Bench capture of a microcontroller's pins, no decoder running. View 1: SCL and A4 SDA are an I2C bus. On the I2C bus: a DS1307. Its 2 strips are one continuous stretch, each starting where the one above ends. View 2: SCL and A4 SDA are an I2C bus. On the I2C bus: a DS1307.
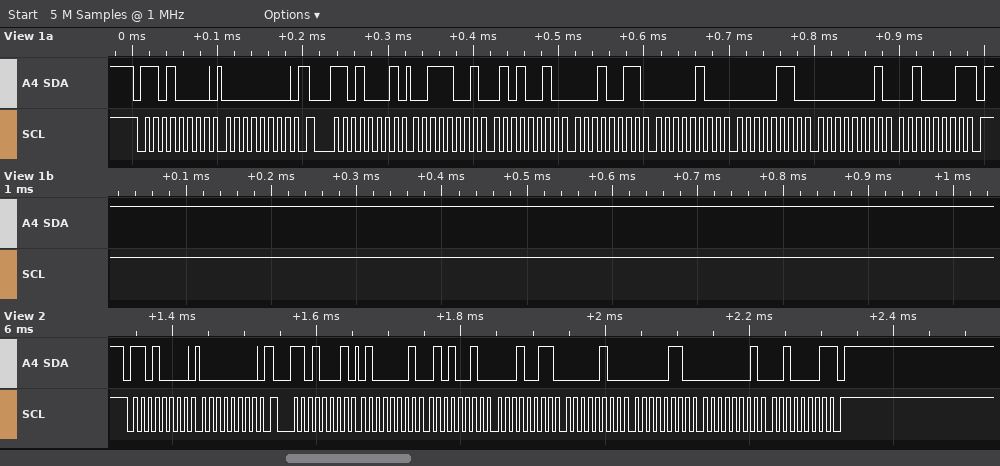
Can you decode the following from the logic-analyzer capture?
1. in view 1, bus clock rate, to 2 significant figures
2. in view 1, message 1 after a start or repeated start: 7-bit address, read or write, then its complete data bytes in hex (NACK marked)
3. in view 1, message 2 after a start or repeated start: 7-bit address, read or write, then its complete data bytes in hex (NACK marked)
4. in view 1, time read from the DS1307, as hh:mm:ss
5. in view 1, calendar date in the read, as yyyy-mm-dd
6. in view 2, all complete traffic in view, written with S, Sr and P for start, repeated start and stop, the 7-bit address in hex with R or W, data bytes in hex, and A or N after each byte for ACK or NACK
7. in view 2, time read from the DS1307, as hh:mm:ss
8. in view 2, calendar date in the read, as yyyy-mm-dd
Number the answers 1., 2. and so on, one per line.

1. 100 kHz
2. 0x68 write: 00
3. 0x68 read: 39 52 13 04 06 01 21 NACK
4. 13:52:39
5. 2021-01-06
6. S 68W A 00 A Sr 68R A 41 A 52 A 13 A 04 A 06 A 01 A 21 N P
7. 13:52:41
8. 2021-01-06
